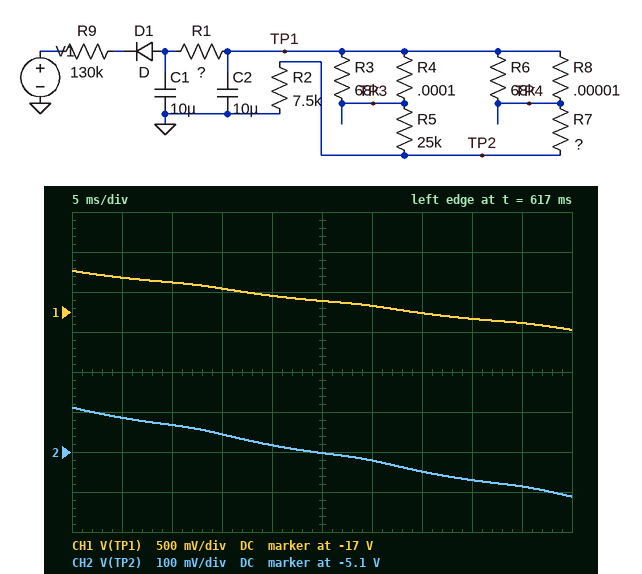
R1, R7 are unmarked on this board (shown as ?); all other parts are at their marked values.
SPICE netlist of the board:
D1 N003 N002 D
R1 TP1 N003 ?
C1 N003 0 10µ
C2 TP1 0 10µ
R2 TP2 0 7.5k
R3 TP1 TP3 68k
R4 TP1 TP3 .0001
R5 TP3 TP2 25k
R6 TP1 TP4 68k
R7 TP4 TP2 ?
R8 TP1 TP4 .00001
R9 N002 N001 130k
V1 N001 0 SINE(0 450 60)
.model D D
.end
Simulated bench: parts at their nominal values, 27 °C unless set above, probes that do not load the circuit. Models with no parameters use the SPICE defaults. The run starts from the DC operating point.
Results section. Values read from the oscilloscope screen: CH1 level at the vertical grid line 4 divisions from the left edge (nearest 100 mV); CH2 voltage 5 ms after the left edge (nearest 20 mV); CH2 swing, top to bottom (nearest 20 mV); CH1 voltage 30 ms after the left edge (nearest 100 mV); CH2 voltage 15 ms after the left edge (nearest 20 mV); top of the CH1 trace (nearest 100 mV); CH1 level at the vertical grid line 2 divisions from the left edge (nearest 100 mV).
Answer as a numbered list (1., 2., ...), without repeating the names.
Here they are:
1. -16.8 V
2. -5.02 V
3. 220 mV
4. -16.9 V
5. -5.06 V
6. -16.5 V
7. -16.6 V
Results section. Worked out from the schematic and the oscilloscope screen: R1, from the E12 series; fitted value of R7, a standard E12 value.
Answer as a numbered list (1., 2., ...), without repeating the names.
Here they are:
1. 10 kΩ
2. 56 kΩ
